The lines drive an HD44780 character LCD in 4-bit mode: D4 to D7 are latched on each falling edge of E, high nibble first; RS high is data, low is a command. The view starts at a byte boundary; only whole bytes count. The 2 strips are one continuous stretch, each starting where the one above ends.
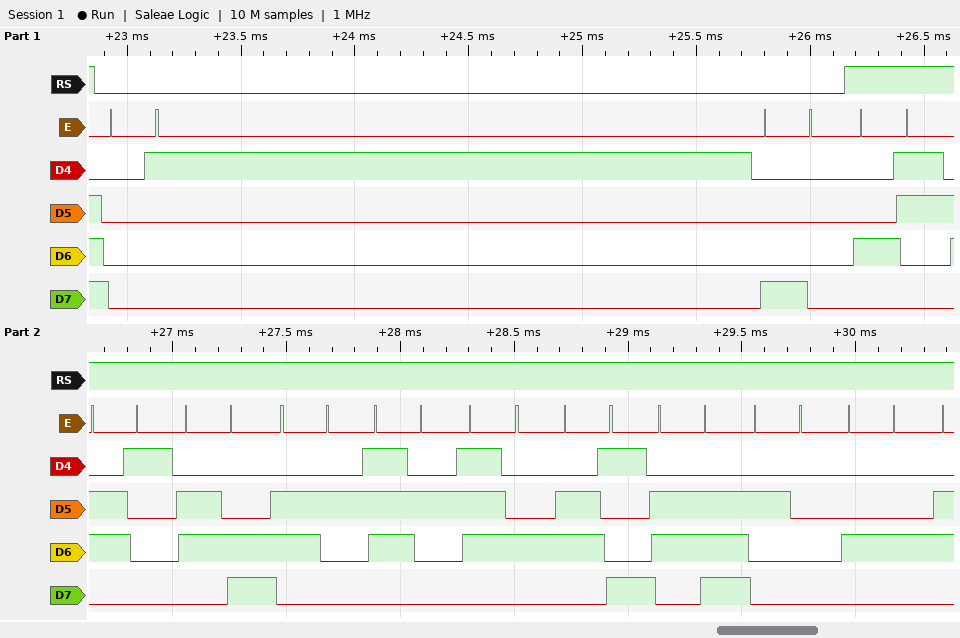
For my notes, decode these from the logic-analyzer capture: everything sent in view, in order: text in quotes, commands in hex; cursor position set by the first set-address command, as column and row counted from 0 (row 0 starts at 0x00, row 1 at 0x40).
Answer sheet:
0x01 0x80 "Calbrtin D"
column 0, row 0
